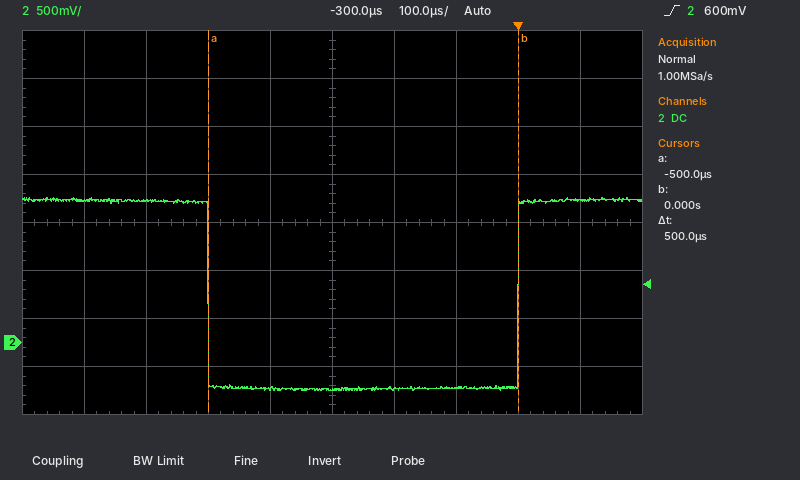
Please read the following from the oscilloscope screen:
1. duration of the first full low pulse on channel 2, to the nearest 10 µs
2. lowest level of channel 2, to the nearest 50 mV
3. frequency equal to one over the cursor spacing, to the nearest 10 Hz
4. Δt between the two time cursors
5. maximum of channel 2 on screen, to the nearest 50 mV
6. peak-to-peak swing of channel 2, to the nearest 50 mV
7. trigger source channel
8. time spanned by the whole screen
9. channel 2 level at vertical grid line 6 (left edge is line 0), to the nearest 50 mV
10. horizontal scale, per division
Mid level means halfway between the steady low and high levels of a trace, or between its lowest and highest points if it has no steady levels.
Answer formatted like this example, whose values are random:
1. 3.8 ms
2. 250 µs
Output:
1. 500 µs
2. -500 mV
3. 2.00 kHz
4. 500 µs
5. 1.50 V
6. 2.00 V
7. channel 2
8. 1 ms
9. -500 mV
10. 100 µs
